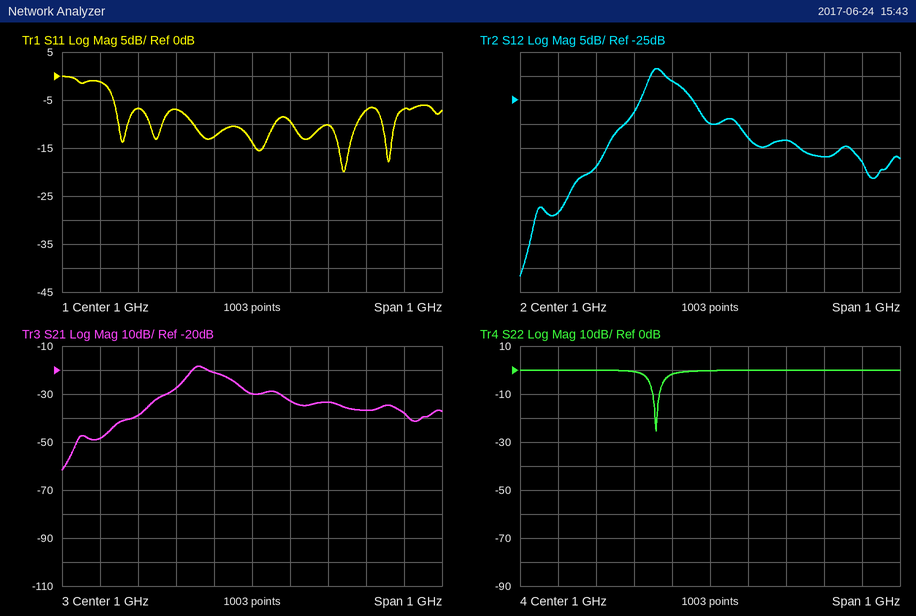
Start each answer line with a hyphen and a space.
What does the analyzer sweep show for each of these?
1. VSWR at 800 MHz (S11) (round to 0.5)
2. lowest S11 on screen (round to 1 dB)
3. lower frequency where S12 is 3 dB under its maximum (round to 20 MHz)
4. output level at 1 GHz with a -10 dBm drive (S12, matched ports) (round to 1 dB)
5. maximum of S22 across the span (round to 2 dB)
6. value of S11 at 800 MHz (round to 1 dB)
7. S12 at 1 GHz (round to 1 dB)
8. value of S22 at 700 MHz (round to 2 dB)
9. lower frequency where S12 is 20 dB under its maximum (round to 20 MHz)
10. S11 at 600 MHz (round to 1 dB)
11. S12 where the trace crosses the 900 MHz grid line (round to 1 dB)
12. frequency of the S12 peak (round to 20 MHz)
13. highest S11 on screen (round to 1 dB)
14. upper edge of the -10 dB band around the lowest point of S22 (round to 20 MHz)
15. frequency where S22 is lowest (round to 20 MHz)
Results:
- 2.5
- -20 dB
- 840 MHz
- -40 dBm
- 0 dB
- -7 dB
- -30 dB
- 0 dB
- 700 MHz
- -1 dB
- -21 dB
- 860 MHz
- 0 dB
- 860 MHz
- 860 MHz
